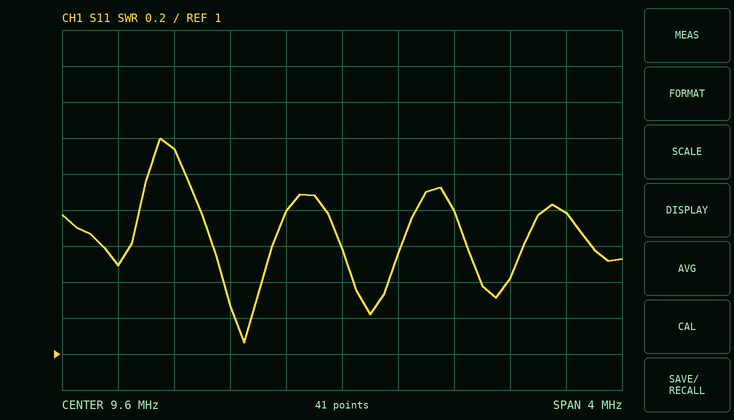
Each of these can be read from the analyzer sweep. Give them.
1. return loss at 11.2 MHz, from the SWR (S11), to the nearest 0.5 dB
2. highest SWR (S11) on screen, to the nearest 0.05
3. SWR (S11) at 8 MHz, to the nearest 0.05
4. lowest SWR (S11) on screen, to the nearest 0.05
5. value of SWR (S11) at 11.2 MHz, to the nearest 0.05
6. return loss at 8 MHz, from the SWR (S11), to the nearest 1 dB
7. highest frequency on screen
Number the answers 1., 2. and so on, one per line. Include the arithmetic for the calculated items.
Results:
1. −20 log10((1.8 − 1)/(1.8 + 1)) ≈ 10.9 dB, so 11.0 dB to the nearest 0.5 dB
2. 2.20
3. 1.50
4. 1.05
5. 1.80
6. −20 log10((1.5 − 1)/(1.5 + 1)) ≈ 14 dB
7. 11.6 MHz
